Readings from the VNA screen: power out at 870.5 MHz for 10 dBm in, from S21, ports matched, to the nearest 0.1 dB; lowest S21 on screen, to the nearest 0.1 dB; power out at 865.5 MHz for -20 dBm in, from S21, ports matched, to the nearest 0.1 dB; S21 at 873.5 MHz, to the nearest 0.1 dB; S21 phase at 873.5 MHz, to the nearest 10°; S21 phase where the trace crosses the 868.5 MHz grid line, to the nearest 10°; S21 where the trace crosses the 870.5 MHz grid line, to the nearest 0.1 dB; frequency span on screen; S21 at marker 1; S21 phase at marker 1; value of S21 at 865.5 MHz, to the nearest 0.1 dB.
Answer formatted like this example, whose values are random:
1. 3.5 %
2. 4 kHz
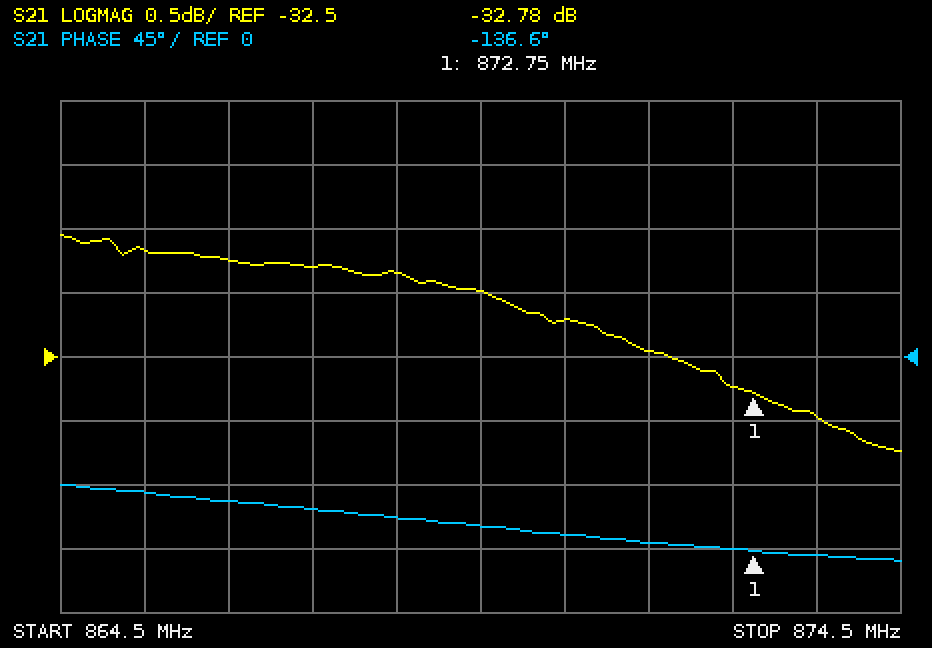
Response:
1. -22.2 dBm
2. -33.2 dB
3. -51.7 dBm
4. -33.0 dB
5. -140°
6. -110°
7. -32.2 dB
8. 10 MHz
9. -32.78 dB
10. -136.6°
11. -31.7 dB
